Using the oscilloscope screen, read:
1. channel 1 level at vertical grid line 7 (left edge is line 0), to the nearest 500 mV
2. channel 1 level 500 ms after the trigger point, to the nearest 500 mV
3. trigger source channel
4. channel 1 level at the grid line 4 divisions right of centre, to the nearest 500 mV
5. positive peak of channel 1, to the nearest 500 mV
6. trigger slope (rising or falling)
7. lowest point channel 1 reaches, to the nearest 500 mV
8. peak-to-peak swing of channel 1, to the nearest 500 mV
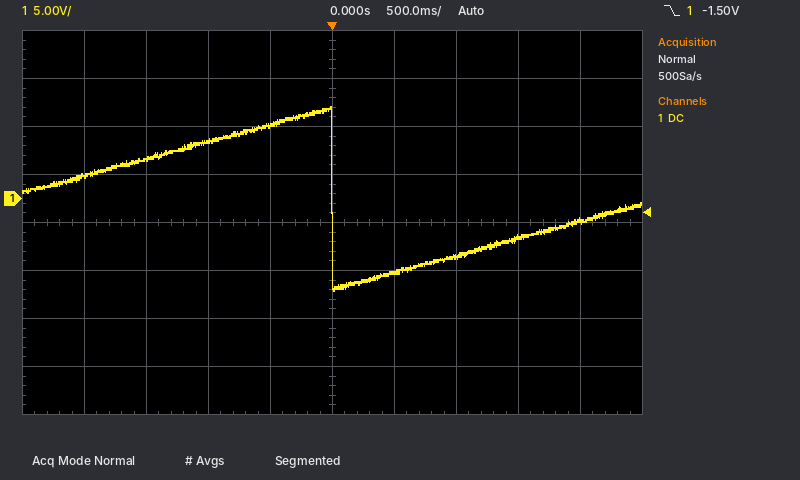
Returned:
-6.0 V
-7.5 V
channel 1
-2.5 V
9.5 V
falling
-9.5 V
19.0 V
